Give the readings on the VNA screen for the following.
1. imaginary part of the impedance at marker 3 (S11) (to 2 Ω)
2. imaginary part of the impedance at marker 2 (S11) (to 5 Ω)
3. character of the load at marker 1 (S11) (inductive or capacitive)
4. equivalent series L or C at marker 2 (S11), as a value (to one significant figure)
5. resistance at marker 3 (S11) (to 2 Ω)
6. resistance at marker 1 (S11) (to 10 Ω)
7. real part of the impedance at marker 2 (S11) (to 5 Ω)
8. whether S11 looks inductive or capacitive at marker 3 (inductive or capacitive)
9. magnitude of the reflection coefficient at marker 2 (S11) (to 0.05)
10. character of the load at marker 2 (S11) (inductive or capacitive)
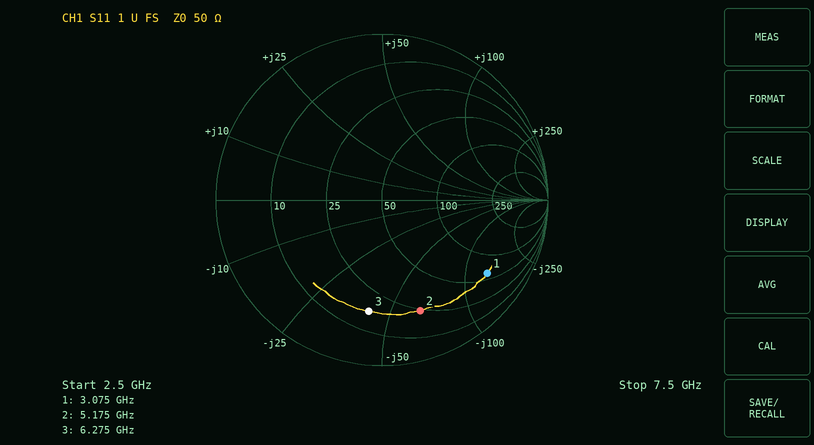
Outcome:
-42 Ω
-65 Ω
capacitive
500 fF
16 Ω
60 Ω
25 Ω
capacitive
0.70
capacitive
